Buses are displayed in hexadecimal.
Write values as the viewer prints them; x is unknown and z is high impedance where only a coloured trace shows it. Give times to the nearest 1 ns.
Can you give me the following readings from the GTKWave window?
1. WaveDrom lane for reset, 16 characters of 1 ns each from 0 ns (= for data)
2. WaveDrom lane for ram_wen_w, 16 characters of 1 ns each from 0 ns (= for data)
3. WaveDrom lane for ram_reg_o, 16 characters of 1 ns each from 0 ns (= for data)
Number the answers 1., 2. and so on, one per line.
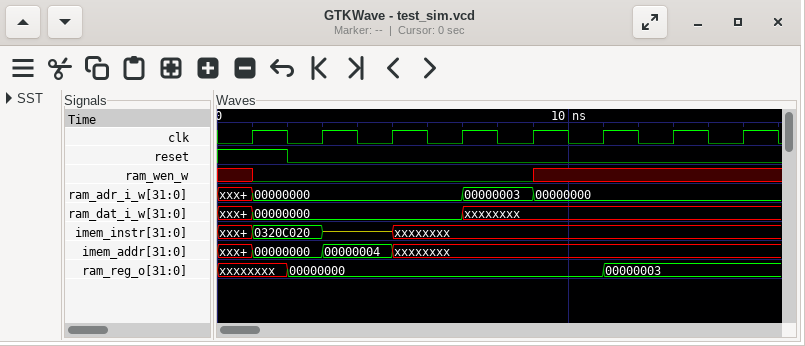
1. {name: 'reset', wave: '1.0.............'}
2. {name: 'ram_wen_w', wave: 'x0.......x......'}
3. {name: 'ram_reg_o', wave: 'x.=........=....', data: '00000000 00000003'}
